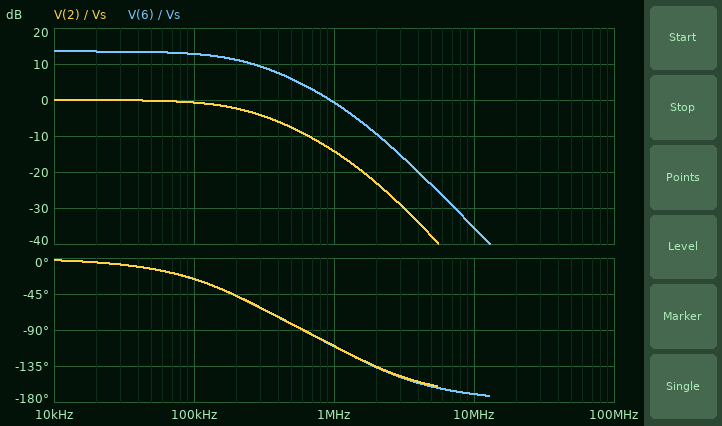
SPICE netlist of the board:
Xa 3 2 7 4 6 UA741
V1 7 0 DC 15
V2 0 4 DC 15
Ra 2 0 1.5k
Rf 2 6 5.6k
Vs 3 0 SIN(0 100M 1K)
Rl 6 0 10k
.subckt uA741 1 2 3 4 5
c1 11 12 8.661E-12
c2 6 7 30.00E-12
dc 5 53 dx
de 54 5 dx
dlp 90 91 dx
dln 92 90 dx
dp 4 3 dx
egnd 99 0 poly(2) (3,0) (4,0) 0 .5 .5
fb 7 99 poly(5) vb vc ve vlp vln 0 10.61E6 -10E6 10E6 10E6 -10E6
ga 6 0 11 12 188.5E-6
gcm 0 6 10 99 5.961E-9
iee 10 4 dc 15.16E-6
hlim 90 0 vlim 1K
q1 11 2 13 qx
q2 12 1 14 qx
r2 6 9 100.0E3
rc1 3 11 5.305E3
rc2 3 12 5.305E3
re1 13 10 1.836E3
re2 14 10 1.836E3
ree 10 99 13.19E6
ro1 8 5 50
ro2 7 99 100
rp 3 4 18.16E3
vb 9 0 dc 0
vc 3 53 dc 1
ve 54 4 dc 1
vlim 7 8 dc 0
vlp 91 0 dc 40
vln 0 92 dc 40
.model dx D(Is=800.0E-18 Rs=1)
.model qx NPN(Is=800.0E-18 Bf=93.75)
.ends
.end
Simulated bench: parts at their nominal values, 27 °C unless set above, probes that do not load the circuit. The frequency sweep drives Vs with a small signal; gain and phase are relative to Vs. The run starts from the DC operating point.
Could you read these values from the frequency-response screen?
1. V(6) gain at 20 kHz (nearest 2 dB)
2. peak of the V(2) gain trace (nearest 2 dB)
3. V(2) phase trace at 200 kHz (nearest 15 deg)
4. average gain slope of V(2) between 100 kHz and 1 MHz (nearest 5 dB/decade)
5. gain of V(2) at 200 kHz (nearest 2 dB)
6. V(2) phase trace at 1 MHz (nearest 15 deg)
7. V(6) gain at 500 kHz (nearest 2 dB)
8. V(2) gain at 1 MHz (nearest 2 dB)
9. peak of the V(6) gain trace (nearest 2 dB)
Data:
14 dB
0 dB
-45 deg
-15 dB/decade
-2 dB
-105 deg
6 dB
-14 dB
14 dB
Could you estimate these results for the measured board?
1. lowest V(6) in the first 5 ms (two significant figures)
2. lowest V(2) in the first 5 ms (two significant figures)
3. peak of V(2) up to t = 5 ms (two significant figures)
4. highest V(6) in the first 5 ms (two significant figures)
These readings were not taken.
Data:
-470 mV
-100 mV
100 mV
470 mV
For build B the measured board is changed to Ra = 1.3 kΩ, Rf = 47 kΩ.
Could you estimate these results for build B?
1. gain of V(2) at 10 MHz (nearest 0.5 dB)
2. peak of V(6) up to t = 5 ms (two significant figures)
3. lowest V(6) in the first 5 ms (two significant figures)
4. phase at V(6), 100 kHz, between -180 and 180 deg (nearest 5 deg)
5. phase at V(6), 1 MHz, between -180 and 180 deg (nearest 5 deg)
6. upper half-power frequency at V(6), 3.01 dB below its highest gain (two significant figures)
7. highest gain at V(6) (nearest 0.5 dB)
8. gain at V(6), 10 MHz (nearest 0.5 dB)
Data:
-61.5 dB
3.7 V
-3.7 V
-80 deg
-120 deg
27 kHz
31.5 dB
-35.5 dB
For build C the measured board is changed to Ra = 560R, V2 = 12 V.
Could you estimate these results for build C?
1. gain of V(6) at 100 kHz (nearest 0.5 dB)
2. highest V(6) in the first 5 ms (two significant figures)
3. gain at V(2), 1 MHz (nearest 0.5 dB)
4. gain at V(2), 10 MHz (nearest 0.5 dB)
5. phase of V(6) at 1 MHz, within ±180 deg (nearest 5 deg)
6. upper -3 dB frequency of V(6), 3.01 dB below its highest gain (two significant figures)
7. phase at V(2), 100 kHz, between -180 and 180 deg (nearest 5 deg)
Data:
17.5 dB
1.1 V
-22.0 dB
-60.0 dB
-115 deg
94 kHz
-50 deg
